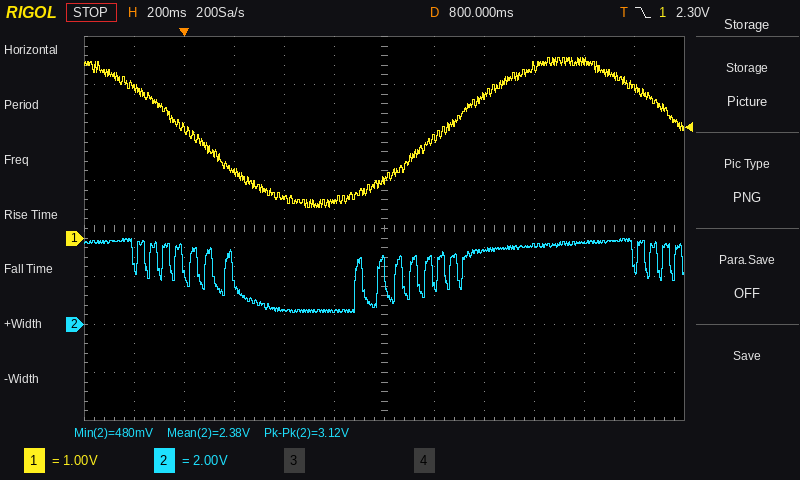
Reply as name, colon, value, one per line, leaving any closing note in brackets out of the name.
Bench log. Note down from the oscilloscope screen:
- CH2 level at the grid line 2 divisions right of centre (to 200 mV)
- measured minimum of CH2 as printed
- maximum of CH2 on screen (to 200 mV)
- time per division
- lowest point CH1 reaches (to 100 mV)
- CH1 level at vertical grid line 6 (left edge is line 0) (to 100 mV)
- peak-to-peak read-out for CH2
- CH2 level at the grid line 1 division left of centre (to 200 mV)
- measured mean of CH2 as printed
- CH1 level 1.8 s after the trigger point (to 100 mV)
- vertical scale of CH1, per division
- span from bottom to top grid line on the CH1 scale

CH2 level at the grid line 2 divisions right of centre: 3.0 V
measured minimum of CH2 as printed: 480 mV
maximum of CH2 on screen: 3.6 V
time per division: 200 ms
lowest point CH1 reaches: 600 mV
CH1 level at vertical grid line 6 (left edge is line 0): 1.2 V
peak-to-peak read-out for CH2: 3.12 V
CH2 level at the grid line 1 division left of centre: 600 mV
measured mean of CH2 as printed: 2.38 V
CH1 level 1.8 s after the trigger point: 3.1 V
vertical scale of CH1, per division: 1 V
span from bottom to top grid line on the CH1 scale: 8 V
